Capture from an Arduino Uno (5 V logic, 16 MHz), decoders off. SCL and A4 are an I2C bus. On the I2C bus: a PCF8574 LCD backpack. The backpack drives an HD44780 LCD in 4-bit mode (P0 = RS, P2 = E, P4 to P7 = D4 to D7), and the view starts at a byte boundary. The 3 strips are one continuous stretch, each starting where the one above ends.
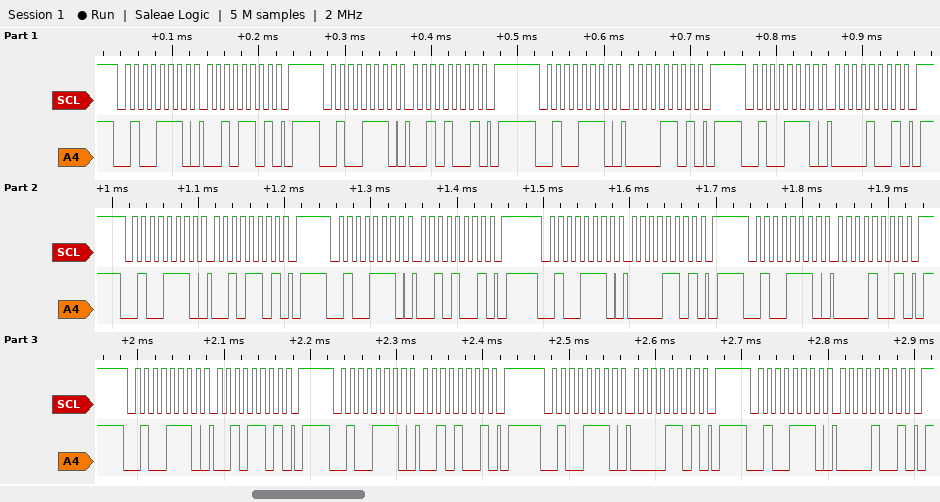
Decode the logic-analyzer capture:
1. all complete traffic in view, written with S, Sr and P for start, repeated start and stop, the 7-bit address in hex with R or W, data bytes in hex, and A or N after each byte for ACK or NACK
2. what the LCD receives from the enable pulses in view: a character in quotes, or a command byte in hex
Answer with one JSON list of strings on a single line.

["S 27W A 2D A P S 27W A 29 A P S 27W A 0D A P S 27W A 09 A P S 27W A 2D A P S 27W A 29 A P S 27W A 0D A P S 27W A 09 A P S 27W A 2D A P S 27W A 29 A P S 27W A 0D A P S 27W A 09 A P", "' ' ' ' ' '"]
